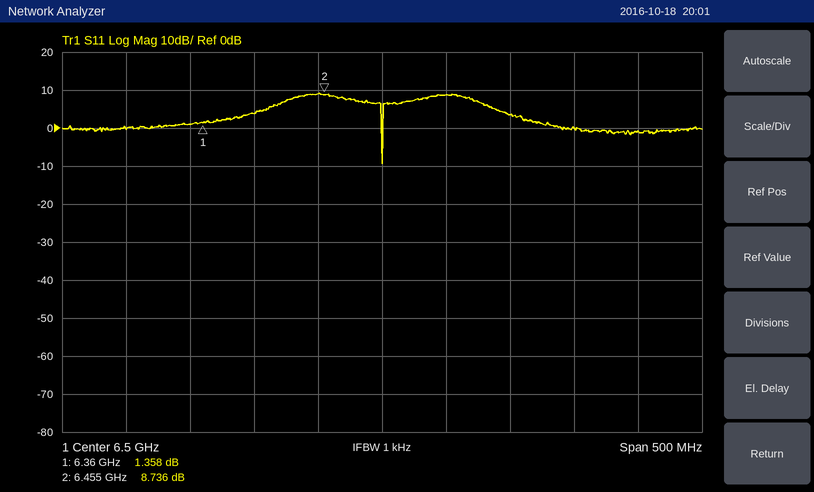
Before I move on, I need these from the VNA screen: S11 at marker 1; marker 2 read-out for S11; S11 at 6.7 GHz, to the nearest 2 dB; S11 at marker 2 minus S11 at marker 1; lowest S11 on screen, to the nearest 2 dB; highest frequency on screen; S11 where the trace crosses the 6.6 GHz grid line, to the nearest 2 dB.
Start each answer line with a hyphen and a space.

- 1.358 dB
- 8.736 dB
- 0 dB
- 7.378 dB
- -10 dB
- 6.75 GHz
- 4 dB
